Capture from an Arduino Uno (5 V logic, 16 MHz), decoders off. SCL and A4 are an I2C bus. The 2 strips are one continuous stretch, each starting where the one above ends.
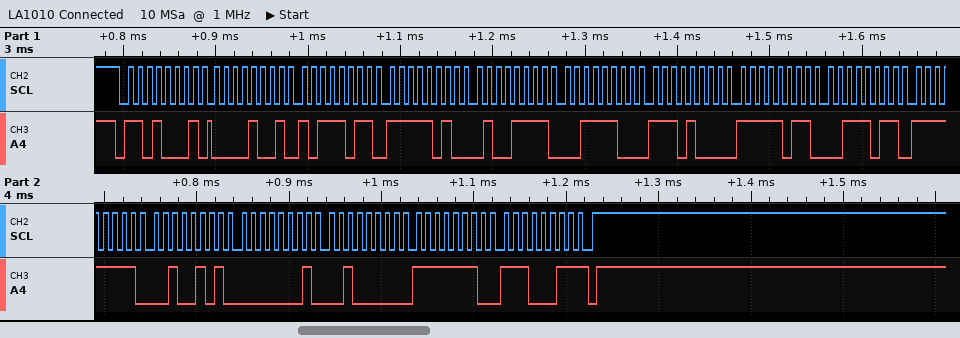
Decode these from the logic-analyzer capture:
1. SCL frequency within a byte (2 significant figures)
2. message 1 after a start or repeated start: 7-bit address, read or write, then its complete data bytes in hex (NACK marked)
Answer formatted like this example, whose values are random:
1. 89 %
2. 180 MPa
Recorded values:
1. 100 kHz
2. 0x68 read: 09 BB FA 4F 3C E8 FB 3B FF 25 01 20 FE E3 NACK
